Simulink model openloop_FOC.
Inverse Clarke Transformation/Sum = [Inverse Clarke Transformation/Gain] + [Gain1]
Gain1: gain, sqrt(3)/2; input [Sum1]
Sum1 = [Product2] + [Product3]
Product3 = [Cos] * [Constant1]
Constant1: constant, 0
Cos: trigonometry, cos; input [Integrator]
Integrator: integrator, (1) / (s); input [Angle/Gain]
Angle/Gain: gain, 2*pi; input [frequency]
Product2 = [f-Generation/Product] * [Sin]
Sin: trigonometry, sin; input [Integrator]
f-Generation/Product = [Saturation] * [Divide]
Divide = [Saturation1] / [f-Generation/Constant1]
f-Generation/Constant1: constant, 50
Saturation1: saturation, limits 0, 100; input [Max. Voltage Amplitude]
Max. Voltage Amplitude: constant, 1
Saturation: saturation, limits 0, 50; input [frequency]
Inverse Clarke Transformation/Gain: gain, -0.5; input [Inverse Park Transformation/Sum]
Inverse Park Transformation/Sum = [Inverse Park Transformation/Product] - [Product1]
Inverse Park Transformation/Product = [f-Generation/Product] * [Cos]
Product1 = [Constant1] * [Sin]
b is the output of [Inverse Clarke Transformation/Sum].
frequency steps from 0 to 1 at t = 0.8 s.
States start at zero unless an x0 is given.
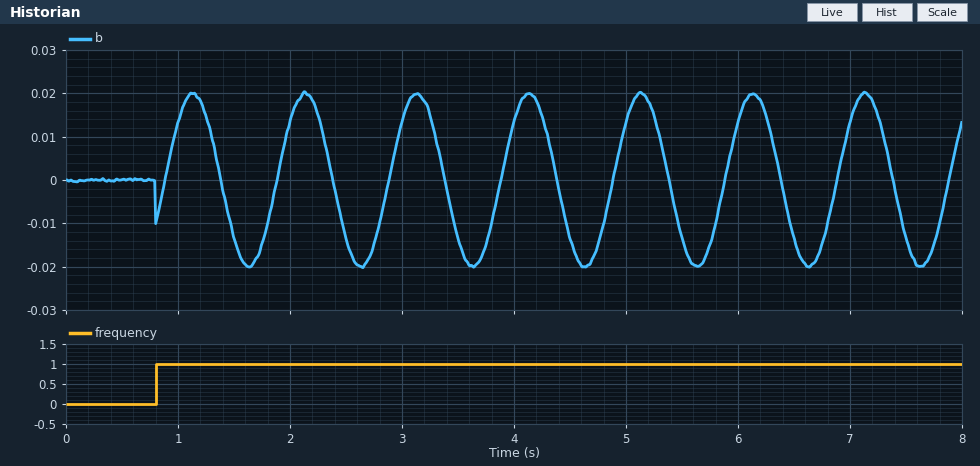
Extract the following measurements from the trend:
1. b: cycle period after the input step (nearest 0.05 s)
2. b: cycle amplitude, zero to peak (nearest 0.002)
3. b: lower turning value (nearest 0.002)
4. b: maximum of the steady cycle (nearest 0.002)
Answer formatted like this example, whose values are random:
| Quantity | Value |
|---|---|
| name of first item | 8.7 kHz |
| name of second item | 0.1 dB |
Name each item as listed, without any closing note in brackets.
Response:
| Quantity | Value |
|---|---|
| b: cycle period after the input step | 1.00 s |
| b: cycle amplitude, zero to peak | 0.020 |
| b: lower turning value | -0.020 |
| b: maximum of the steady cycle | 0.020 |
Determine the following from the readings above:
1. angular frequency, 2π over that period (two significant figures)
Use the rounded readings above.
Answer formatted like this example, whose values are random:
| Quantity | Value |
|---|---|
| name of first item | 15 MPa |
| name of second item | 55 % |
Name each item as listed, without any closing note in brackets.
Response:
| Quantity | Value |
|---|---|
| angular frequency, 2π over that period | 6.3 rad/s |
